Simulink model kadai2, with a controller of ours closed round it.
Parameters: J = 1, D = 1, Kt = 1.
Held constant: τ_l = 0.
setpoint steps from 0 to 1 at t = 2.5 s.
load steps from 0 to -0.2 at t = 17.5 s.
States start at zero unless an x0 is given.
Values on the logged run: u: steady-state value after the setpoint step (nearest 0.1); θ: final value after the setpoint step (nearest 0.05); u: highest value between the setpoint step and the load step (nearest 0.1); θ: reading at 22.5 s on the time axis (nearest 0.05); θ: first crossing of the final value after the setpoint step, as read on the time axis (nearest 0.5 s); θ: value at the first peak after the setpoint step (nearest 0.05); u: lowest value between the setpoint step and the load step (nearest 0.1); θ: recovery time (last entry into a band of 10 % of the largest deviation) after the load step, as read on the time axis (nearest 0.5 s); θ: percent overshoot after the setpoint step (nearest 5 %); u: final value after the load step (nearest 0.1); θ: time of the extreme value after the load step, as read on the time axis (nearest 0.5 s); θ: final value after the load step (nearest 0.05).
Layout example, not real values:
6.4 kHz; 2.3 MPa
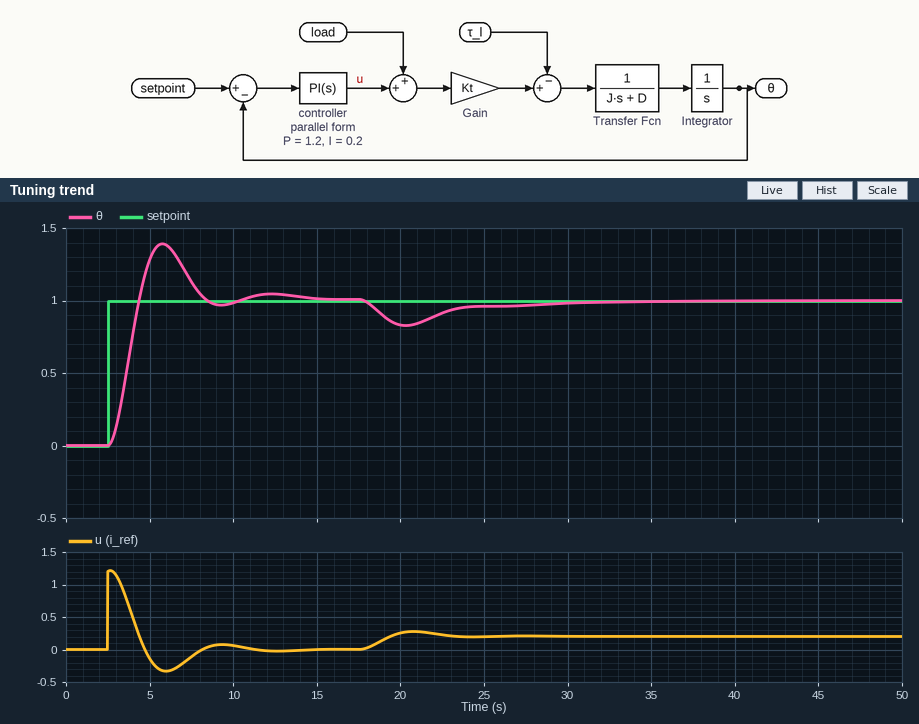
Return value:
0.0; 1.00; 1.2; 0.90; 4.5 s; 1.40; -0.3; 30.0 s; 40 %; 0.2; 20.5 s; 1.00
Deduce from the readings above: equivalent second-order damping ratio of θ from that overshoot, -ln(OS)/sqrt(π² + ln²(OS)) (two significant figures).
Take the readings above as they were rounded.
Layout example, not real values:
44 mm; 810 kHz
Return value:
0.28
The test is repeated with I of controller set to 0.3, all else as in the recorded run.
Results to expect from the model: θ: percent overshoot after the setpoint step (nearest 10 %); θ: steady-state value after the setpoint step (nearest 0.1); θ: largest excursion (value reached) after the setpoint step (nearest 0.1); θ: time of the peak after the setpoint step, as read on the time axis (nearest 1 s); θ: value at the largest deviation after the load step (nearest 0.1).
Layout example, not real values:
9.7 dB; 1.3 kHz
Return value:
50 %; 1.0; 1.5; 6 s; 0.8
